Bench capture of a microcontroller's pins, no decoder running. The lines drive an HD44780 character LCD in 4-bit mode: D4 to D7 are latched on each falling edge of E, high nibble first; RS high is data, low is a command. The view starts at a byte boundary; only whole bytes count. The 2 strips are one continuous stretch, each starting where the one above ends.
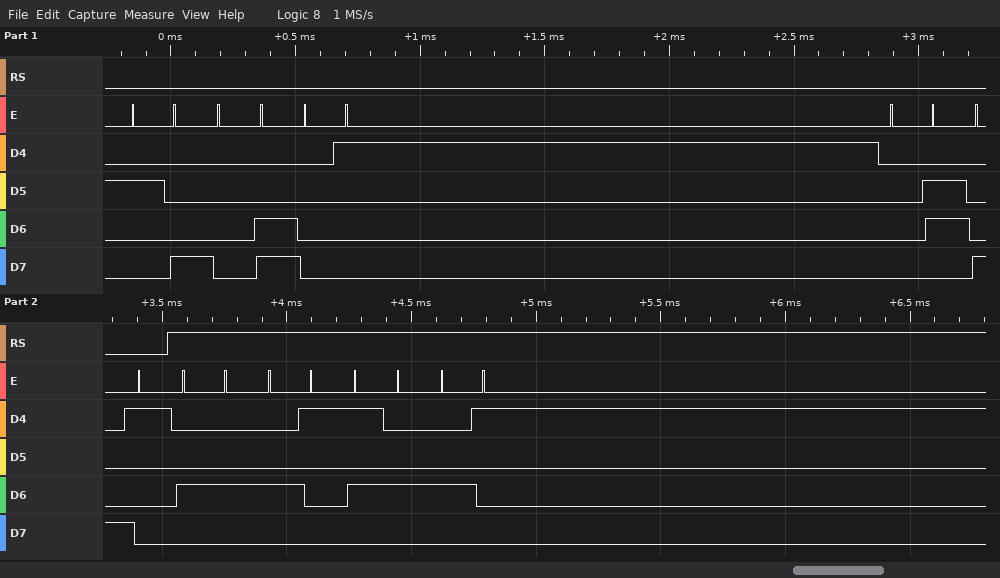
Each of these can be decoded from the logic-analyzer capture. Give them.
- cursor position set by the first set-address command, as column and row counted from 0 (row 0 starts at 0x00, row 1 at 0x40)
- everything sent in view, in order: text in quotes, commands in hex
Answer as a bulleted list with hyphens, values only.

- column 1, row 0
- 0x28 0x0C 0x01 0x06 0x81 "DATA"
